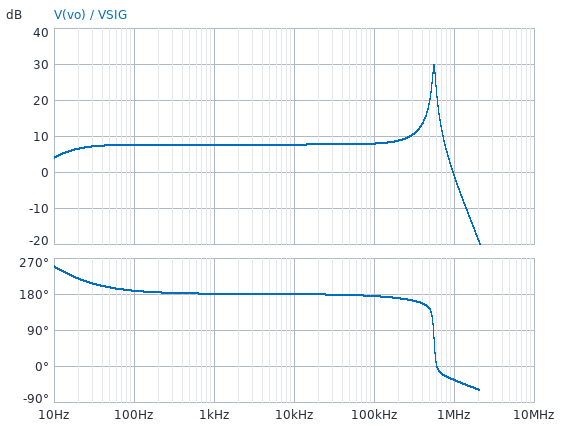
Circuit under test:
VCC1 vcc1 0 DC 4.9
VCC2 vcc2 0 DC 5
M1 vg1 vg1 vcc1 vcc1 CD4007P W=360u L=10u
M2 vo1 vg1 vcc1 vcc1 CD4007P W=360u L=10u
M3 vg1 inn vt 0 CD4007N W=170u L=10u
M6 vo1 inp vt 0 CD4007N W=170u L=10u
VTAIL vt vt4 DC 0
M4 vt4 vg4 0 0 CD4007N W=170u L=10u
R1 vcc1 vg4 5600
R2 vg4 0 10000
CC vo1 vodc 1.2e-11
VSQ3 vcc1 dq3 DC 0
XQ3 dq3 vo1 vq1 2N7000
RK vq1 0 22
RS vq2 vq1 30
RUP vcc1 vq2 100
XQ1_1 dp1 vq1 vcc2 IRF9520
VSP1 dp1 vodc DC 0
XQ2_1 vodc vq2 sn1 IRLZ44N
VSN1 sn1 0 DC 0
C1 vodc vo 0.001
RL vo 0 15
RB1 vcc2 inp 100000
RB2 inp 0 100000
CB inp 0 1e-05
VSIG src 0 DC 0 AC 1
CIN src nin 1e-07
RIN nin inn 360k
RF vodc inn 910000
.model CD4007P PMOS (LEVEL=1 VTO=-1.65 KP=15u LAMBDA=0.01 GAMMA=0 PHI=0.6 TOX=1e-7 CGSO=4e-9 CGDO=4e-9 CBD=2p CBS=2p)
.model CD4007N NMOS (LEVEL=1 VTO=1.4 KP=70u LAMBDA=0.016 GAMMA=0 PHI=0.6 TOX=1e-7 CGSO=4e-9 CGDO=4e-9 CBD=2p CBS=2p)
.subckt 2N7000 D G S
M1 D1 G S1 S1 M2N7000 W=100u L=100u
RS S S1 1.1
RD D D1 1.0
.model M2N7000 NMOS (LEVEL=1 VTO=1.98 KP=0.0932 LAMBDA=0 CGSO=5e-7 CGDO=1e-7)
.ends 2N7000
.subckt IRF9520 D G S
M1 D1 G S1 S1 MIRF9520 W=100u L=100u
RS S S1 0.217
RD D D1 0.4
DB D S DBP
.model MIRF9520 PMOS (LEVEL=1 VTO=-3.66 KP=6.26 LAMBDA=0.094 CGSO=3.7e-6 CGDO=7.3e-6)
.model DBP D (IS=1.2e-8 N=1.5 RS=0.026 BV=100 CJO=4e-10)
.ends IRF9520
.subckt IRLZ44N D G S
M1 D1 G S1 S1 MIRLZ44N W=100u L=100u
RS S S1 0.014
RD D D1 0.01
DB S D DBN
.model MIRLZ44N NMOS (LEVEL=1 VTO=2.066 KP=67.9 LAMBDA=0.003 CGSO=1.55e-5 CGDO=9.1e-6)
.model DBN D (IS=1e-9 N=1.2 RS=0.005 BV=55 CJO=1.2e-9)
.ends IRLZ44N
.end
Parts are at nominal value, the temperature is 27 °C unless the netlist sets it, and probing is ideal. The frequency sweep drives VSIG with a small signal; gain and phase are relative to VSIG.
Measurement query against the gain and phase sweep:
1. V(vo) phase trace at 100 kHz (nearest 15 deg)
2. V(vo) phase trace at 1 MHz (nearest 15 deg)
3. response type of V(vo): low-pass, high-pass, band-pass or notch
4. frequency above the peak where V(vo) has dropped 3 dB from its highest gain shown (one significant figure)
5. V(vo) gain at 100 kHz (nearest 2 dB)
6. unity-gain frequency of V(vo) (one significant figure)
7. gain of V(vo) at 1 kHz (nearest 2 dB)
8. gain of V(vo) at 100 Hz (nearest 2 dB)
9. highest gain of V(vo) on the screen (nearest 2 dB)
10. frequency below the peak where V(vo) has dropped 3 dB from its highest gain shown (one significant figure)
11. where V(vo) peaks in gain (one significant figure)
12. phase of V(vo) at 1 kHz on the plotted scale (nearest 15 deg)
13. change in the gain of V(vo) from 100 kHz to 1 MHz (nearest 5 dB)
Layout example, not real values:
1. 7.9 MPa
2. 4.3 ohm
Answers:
1. 180 deg
2. -30 deg
3. band-pass
4. 600 kHz
5. 8 dB
6. 1 MHz
7. 8 dB
8. 8 dB
9. 30 dB
10. 500 kHz
11. 600 kHz
12. 180 deg
13. -10 dB
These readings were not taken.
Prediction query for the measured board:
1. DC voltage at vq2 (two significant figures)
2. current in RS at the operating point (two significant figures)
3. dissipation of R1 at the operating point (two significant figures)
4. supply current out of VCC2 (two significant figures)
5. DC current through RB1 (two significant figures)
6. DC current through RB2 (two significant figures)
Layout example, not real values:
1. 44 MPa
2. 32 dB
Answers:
1. 2.1 V
2. 28 mA
3. 550 µW
4. 26 mA
5. 25 µA
6. 25 µA
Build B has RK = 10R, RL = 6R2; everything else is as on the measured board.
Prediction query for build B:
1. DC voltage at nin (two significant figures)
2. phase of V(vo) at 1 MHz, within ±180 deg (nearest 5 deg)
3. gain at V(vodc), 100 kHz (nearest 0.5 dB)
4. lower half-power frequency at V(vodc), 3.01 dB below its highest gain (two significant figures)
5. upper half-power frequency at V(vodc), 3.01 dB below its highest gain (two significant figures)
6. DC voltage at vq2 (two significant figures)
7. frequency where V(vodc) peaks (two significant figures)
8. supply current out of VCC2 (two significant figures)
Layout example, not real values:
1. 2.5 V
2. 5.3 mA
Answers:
1. 3.6 V
2. 20 deg
3. -9.0 dB
4. 2.2 Hz
5. 8.2 Hz
6. 2.1 V
7. 4.2 Hz
8. 25 mA
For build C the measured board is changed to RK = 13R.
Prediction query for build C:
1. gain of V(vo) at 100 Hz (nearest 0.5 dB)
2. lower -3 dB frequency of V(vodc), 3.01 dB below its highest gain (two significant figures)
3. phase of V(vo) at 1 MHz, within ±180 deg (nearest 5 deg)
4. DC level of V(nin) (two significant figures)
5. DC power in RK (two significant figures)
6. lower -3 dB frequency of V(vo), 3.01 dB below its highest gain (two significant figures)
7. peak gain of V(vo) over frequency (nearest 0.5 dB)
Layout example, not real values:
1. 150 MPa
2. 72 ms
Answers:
1. 6.0 dB
2. 4.4 Hz
3. 0 deg
4. 2.8 V
5. 120 mW
6. 18 Hz
7. 8.0 dB
